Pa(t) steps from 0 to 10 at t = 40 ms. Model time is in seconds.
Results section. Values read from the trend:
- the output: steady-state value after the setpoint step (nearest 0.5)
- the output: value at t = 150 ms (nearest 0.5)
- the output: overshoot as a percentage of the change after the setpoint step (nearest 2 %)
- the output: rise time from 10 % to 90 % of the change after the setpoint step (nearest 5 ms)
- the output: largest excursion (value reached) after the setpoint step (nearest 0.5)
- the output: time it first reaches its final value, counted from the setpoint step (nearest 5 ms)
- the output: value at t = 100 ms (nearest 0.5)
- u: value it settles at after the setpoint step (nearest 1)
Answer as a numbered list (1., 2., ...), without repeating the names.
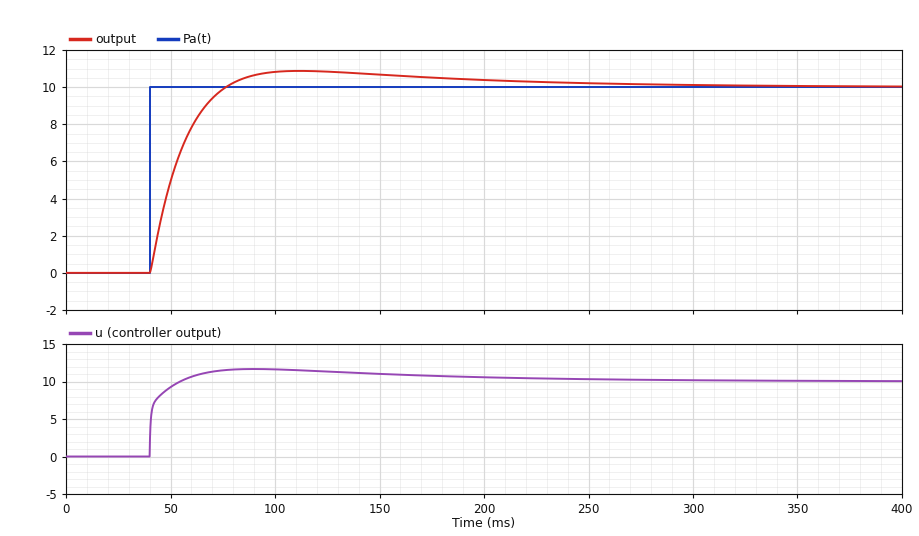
1. 10.0
2. 10.5
3. 8 %
4. 25 ms
5. 11.0
6. 35 ms
7. 11.0
8. 10
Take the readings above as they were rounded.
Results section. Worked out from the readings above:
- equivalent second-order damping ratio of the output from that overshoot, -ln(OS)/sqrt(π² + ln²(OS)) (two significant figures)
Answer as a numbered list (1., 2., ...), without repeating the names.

1. 0.63
